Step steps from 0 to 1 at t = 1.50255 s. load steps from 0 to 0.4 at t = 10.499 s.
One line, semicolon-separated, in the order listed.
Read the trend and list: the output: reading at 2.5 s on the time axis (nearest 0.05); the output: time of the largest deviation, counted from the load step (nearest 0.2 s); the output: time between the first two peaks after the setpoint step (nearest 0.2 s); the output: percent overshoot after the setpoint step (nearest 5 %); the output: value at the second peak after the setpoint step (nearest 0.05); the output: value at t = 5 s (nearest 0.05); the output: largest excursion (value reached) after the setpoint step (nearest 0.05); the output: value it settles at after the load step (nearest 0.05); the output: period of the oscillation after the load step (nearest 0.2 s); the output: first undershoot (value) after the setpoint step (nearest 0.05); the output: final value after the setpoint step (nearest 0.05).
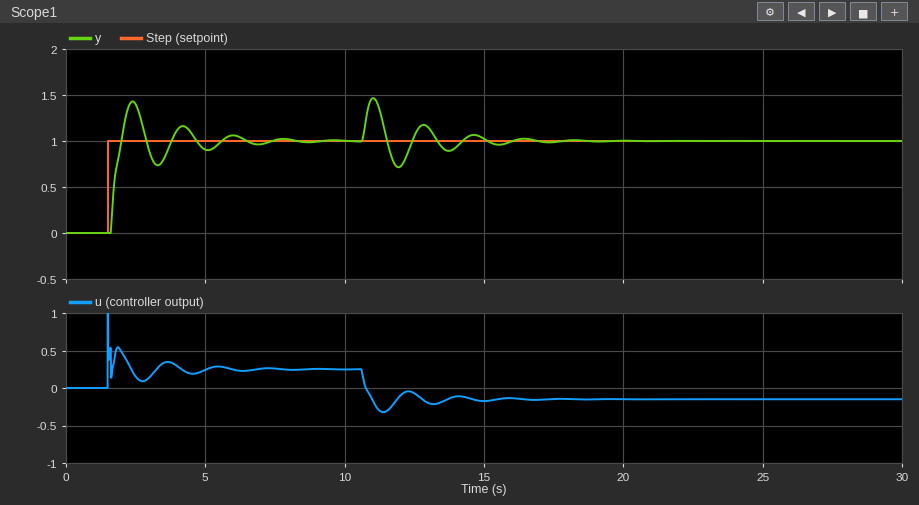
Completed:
1.40; 0.6 s; 1.8 s; 45 %; 1.15; 0.90; 1.45; 1.00; 1.8 s; 0.75; 1.00
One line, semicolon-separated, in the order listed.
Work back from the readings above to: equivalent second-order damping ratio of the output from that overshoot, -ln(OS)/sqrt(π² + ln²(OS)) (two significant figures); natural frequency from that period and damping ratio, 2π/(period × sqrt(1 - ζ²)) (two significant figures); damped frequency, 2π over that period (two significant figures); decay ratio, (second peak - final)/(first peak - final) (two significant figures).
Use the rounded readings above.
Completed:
0.25; 3.6 rad/s; 3.5 rad/s; 0.33
